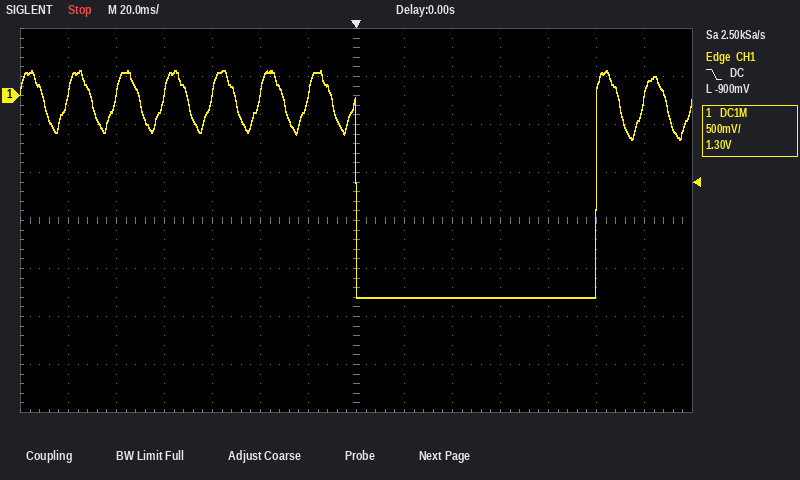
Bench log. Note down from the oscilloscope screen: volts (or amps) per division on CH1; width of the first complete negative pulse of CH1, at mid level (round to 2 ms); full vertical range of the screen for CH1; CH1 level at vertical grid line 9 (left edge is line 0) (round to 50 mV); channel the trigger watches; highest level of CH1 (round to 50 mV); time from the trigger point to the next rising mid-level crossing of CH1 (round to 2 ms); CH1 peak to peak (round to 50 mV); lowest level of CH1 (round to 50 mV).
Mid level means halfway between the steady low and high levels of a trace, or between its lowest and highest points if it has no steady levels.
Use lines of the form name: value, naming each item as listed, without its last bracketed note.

volts (or amps) per division on CH1: 500 mV
width of the first complete negative pulse of CH1, at mid level: 100 ms
full vertical range of the screen for CH1: 4 V
CH1 level at vertical grid line 9 (left edge is line 0): -2.10 V
channel the trigger watches: CH1
highest level of CH1: 250 mV
time from the trigger point to the next rising mid-level crossing of CH1: 100 ms
CH1 peak to peak: 2.35 V
lowest level of CH1: -2.10 V
